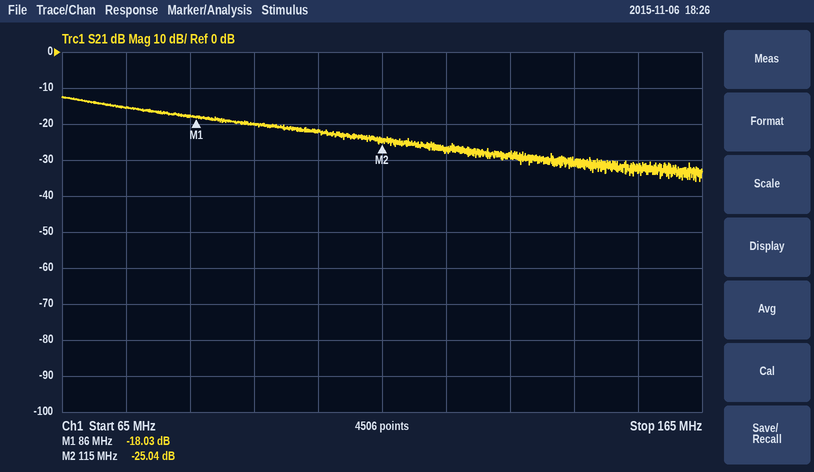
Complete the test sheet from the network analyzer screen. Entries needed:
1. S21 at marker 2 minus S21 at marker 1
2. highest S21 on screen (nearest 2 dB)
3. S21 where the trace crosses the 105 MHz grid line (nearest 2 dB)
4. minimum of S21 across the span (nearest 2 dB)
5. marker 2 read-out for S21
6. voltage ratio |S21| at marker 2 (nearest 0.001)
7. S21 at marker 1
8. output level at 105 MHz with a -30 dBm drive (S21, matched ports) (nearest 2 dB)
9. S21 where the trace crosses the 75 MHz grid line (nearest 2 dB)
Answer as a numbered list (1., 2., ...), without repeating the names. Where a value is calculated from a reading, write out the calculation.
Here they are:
1. -25.04 − (-18.03) = -7.01 dB
2. -12 dB
3. -22 dB
4. -36 dB
5. -25.04 dB
6. 10^(-25.04/20) ≈ 0.056
7. -18.03 dB
8. -30 dBm + (-22 dB) = -52 dBm
9. -16 dB
